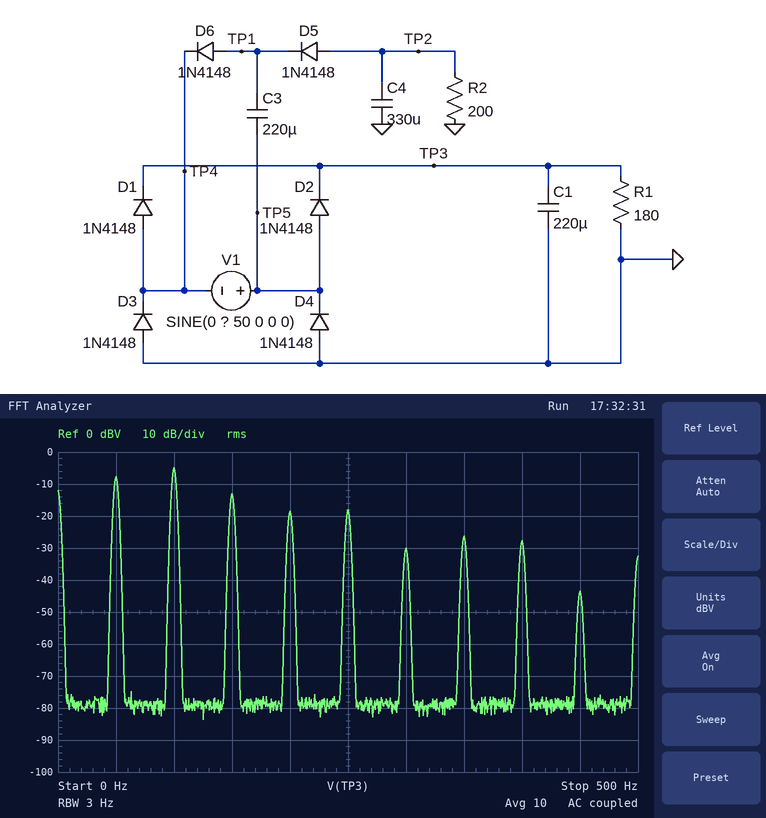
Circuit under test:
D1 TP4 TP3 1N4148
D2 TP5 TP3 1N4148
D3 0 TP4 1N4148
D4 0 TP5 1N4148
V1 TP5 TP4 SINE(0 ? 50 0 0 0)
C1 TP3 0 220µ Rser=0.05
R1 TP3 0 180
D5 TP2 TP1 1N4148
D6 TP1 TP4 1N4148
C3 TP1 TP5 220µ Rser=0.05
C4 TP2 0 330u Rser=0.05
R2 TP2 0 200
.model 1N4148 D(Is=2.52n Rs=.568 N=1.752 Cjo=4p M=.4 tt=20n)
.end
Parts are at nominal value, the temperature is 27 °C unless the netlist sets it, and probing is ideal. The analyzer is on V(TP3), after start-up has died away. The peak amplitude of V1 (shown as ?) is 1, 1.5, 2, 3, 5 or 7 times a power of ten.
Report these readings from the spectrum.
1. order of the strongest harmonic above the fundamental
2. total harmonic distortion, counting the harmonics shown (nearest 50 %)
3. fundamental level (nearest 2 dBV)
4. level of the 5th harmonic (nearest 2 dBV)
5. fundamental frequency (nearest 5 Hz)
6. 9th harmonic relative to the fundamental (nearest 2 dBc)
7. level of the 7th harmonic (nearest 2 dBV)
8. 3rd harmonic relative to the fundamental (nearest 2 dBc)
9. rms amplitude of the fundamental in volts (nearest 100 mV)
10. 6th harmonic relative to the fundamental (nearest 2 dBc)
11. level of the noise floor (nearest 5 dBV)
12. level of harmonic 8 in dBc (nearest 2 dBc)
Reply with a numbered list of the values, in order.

1. 2
2. 150 %
3. -8 dBV
4. -18 dBV
5. 50 Hz
6. -36 dBc
7. -26 dBV
8. -6 dBc
9. 400 mV
10. -22 dBc
11. -80 dBV
12. -20 dBc
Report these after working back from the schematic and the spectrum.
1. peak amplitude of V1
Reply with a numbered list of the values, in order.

1. 15 V
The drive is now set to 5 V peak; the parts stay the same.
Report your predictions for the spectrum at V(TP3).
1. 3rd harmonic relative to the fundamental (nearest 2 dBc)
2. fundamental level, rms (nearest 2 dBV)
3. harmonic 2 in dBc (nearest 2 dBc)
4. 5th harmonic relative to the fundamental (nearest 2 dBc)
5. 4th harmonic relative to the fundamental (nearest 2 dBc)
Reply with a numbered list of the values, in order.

1. -8 dBc
2. -16 dBV
3. 0 dBc
4. -14 dBc
5. -14 dBc
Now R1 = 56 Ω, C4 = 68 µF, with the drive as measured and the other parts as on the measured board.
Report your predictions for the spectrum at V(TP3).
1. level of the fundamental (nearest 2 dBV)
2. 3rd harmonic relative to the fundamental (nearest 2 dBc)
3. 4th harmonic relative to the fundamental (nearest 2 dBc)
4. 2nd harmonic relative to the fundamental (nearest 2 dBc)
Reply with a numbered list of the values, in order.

1. -12 dBV
2. -2 dBc
3. 4 dBc
4. 16 dBc
